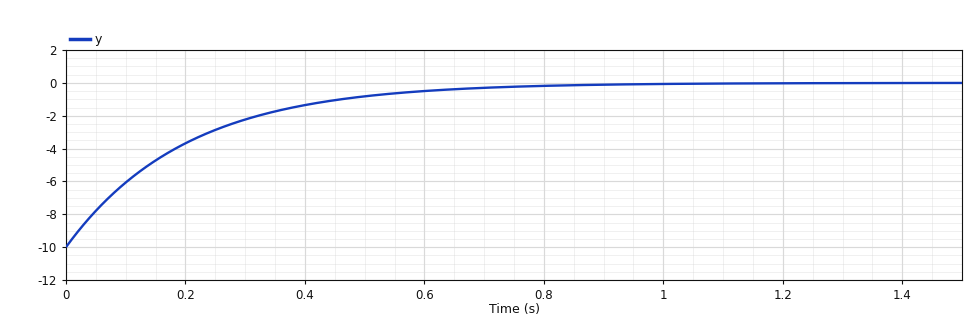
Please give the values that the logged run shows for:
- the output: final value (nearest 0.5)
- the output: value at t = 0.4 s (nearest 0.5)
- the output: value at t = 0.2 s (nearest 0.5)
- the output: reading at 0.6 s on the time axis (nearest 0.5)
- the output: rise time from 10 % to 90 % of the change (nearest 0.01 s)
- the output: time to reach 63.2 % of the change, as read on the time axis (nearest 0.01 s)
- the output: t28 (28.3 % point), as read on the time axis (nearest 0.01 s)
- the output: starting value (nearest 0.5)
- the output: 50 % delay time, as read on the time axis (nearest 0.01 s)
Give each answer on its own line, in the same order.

0.0
-1.5
-3.5
-0.5
0.44 s
0.20 s
0.07 s
-10.0
0.14 s
